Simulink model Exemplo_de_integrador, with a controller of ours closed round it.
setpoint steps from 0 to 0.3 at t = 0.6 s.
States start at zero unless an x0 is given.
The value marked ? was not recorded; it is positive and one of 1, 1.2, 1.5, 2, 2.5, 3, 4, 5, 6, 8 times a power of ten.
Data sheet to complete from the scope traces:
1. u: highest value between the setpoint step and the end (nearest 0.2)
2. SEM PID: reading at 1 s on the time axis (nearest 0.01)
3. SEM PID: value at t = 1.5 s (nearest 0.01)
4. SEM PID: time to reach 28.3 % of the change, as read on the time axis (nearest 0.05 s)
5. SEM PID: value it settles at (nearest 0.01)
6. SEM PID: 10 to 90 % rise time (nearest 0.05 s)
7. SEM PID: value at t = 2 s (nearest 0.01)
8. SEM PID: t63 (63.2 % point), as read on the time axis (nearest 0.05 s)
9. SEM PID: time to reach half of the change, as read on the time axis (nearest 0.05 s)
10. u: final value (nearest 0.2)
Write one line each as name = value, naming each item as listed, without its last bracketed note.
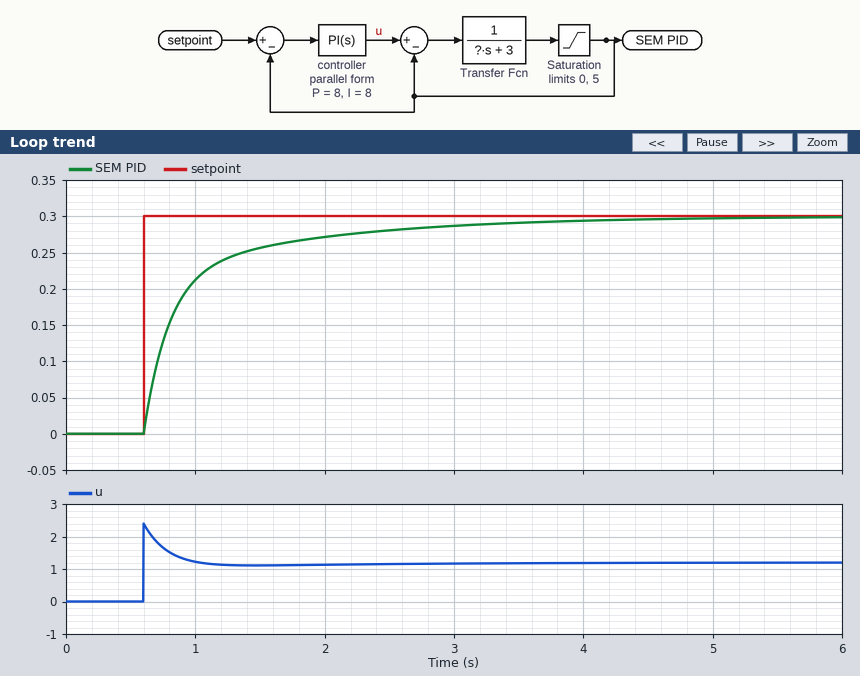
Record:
u: highest value between the setpoint step and the end = 2.4
SEM PID: reading at 1 s on the time axis = 0.21
SEM PID: value at t = 1.5 s = 0.26
SEM PID: time to reach 28.3 % of the change, as read on the time axis = 0.70 s
SEM PID: value it settles at = 0.30
SEM PID: 10 to 90 % rise time = 1.30 s
SEM PID: value at t = 2 s = 0.27
SEM PID: t63 (63.2 % point), as read on the time axis = 0.90 s
SEM PID: time to reach half of the change, as read on the time axis = 0.80 s
u: final value = 1.2
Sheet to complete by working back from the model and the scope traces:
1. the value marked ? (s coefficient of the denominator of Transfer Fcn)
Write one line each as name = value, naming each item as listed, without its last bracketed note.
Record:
the value marked ? = 2
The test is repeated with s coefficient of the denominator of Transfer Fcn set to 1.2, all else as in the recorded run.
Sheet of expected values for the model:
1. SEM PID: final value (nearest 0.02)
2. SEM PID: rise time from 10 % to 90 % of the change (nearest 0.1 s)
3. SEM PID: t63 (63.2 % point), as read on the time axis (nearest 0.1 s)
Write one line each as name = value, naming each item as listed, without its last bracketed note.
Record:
SEM PID: final value = 0.30
SEM PID: rise time from 10 % to 90 % of the change = 1.5 s
SEM PID: t63 (63.2 % point), as read on the time axis = 0.8 s
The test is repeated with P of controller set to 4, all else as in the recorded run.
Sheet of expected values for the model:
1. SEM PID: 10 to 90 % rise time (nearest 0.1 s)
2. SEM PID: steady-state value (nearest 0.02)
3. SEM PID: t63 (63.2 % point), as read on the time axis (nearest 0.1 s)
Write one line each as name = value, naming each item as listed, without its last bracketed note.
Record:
SEM PID: 10 to 90 % rise time = 1.1 s
SEM PID: steady-state value = 0.30
SEM PID: t63 (63.2 % point), as read on the time axis = 1.1 s
